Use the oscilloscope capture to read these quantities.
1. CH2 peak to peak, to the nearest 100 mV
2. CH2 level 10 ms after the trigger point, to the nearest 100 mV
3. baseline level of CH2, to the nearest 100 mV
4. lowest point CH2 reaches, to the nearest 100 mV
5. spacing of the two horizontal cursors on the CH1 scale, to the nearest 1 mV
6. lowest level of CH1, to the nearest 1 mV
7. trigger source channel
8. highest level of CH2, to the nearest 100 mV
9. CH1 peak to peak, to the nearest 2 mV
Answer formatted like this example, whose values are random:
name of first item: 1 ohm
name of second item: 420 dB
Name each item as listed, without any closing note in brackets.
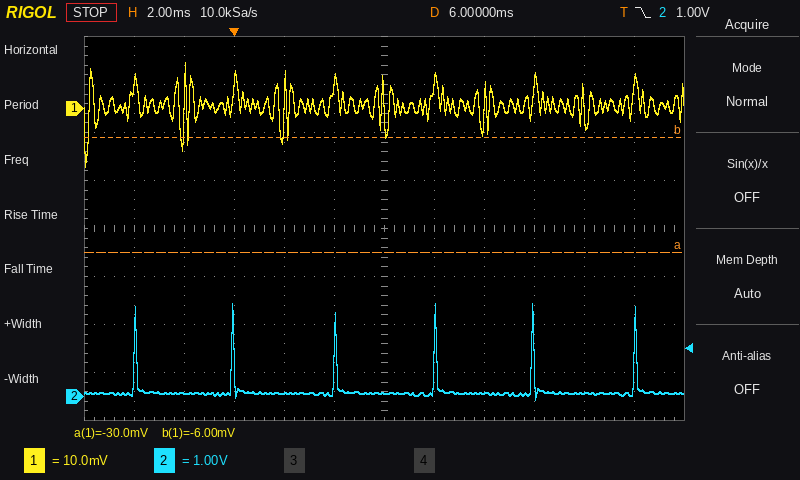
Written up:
CH2 peak to peak, to the nearest 100 mV: 2.0 V
CH2 level 10 ms after the trigger point, to the nearest 100 mV: 100 mV
baseline level of CH2, to the nearest 100 mV: 100 mV
lowest point CH2 reaches, to the nearest 100 mV: -100 mV
spacing of the two horizontal cursors on the CH1 scale, to the nearest 1 mV: 24 mV
lowest level of CH1, to the nearest 1 mV: -12 mV
trigger source channel: CH2
highest level of CH2, to the nearest 100 mV: 1.9 V
CH1 peak to peak, to the nearest 2 mV: 22 mV
